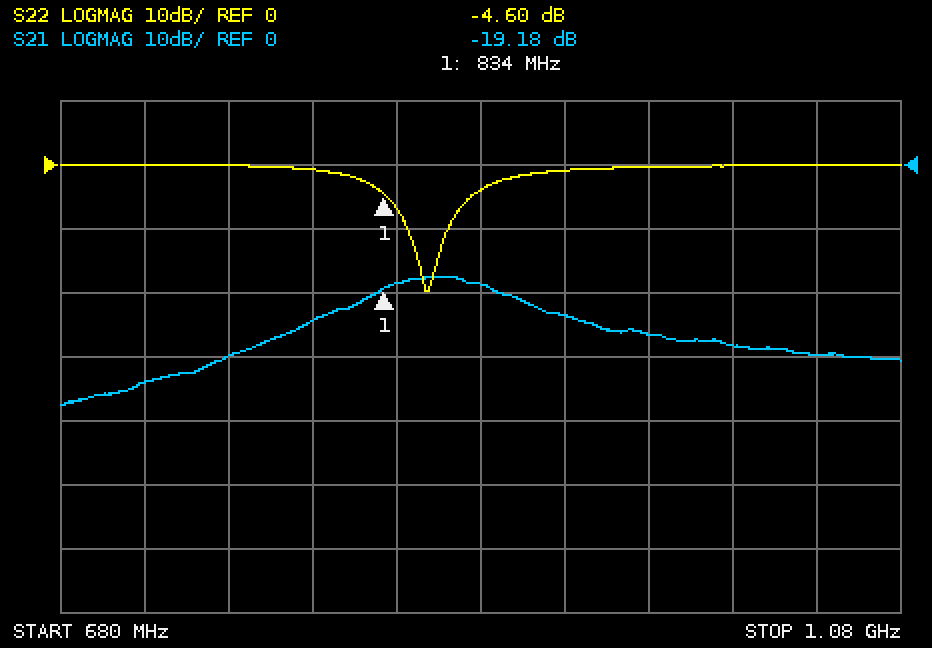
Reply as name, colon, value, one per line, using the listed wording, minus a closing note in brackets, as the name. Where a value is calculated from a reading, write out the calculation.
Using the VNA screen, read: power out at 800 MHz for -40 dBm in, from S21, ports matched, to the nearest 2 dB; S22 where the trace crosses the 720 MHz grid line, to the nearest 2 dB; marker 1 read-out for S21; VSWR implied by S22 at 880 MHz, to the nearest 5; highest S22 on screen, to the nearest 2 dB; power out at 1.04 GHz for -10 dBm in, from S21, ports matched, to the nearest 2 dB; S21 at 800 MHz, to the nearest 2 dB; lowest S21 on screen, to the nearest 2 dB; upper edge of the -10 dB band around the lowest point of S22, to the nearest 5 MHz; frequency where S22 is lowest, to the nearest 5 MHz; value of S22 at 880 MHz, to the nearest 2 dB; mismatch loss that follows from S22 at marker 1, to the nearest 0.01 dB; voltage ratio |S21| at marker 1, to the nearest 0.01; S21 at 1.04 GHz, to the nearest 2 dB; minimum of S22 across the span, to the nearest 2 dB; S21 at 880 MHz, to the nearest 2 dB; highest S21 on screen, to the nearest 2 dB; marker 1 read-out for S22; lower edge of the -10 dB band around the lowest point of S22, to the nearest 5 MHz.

power out at 800 MHz for -40 dBm in, from S21, ports matched, to the nearest 2 dB: -40 dBm + (-24 dB) = -64 dBm
S22 where the trace crosses the 720 MHz grid line, to the nearest 2 dB: 0 dB
marker 1 read-out for S21: -19.18 dB
VSWR implied by S22 at 880 MHz, to the nearest 5: |Γ| = 10^(-4/20) = 0.6310; VSWR = (1 + 0.6310)/(1 − 0.6310) ≈ 4.42, so 5 to the nearest 5
highest S22 on screen, to the nearest 2 dB: 0 dB
power out at 1.04 GHz for -10 dBm in, from S21, ports matched, to the nearest 2 dB: -10 dBm + (-30 dB) = -40 dBm
S21 at 800 MHz, to the nearest 2 dB: -24 dB
lowest S21 on screen, to the nearest 2 dB: -38 dB
upper edge of the -10 dB band around the lowest point of S22, to the nearest 5 MHz: 865 MHz
frequency where S22 is lowest, to the nearest 5 MHz: 855 MHz
value of S22 at 880 MHz, to the nearest 2 dB: -4 dB
mismatch loss that follows from S22 at marker 1, to the nearest 0.01 dB: −10 log10(1 − 10^(-4.6/10)) ≈ 1.85 dB
voltage ratio |S21| at marker 1, to the nearest 0.01: 10^(-19.18/20) ≈ 0.11
S21 at 1.04 GHz, to the nearest 2 dB: -30 dB
minimum of S22 across the span, to the nearest 2 dB: -20 dB
S21 at 880 MHz, to the nearest 2 dB: -18 dB
highest S21 on screen, to the nearest 2 dB: -18 dB
marker 1 read-out for S22: -4.60 dB
lower edge of the -10 dB band around the lowest point of S22, to the nearest 5 MHz: 845 MHz
